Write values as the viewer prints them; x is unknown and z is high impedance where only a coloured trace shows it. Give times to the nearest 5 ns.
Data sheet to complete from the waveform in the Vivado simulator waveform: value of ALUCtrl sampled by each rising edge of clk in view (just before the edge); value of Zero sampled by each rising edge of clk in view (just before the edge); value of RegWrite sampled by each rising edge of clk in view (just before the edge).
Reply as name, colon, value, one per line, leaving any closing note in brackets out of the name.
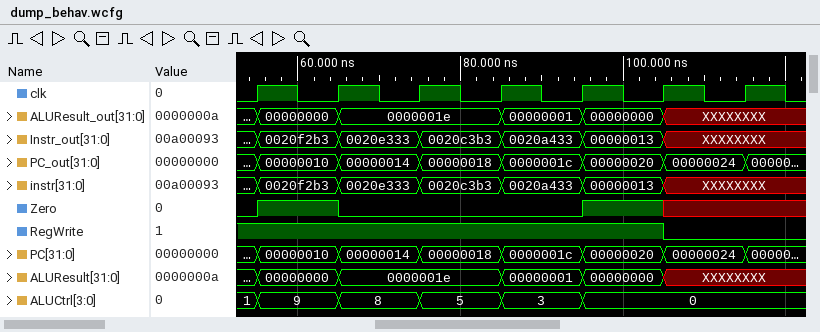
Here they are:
value of ALUCtrl sampled by each rising edge of clk in view: 1, 9, 8, 5, 3, 0, 0
value of Zero sampled by each rising edge of clk in view: 0 1 0 0 0 1 x
value of RegWrite sampled by each rising edge of clk in view: 1 1 1 1 1 1 0
